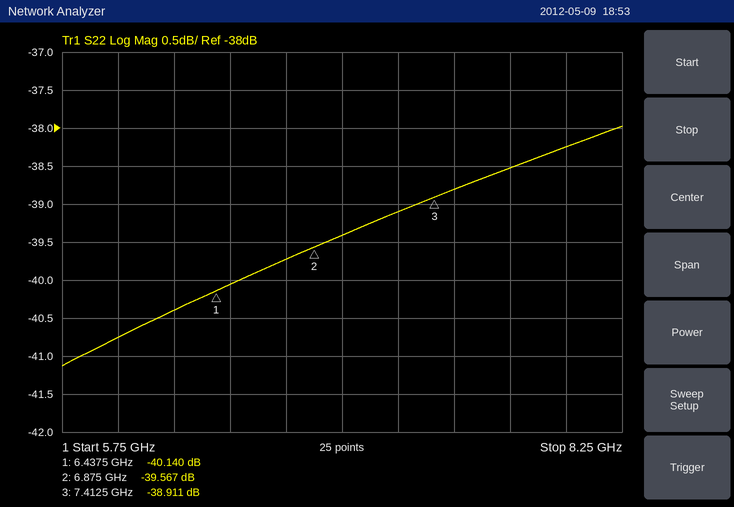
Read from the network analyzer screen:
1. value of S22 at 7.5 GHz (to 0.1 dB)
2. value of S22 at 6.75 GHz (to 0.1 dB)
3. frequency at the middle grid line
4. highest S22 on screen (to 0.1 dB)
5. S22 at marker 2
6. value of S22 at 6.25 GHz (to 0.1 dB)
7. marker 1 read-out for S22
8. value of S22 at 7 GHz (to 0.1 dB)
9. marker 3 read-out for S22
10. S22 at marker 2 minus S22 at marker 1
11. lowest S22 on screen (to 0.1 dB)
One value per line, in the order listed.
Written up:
-38.8 dB
-39.7 dB
7 GHz
-38.0 dB
-39.567 dB
-40.4 dB
-40.140 dB
-39.4 dB
-38.911 dB
0.573 dB
-41.1 dB
